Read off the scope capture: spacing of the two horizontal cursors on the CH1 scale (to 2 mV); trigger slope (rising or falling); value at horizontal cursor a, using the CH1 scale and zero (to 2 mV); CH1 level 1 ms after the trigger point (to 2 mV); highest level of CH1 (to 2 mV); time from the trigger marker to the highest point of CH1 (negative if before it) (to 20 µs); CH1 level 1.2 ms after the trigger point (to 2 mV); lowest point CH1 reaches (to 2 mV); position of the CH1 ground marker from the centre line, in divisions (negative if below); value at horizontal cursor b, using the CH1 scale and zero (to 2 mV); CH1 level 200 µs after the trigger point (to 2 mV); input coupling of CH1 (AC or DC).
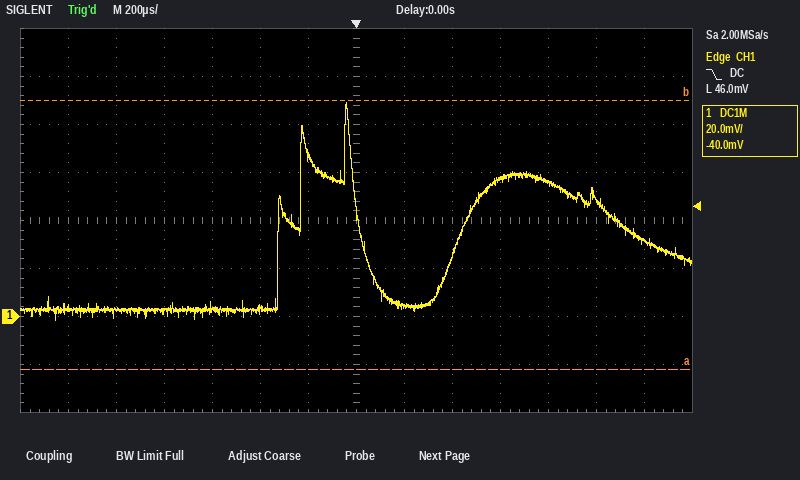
112 mV
falling
-22 mV
48 mV
90 mV
-40 µs
32 mV
-2 mV
-2.0 div
90 mV
4 mV
DC
